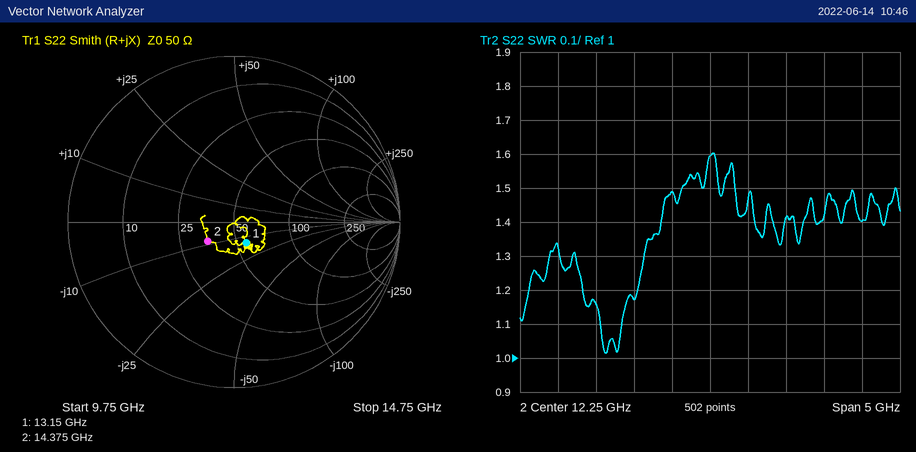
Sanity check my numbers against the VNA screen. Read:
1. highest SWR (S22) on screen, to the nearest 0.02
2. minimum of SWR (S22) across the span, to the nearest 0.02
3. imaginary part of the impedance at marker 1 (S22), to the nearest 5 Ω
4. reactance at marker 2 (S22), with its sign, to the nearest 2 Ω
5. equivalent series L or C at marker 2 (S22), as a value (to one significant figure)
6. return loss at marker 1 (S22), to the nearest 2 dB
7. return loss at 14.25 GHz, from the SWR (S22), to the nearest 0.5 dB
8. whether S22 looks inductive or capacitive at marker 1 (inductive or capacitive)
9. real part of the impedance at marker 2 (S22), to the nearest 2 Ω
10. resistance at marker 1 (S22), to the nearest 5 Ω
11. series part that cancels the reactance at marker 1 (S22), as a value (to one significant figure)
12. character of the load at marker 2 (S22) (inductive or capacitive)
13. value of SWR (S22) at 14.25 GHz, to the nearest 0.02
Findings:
1.60
1.02
-15 Ω
-8 Ω
1 pF
16 dB
15.5 dB
capacitive
36 Ω
55 Ω
200 pH
capacitive
1.40
